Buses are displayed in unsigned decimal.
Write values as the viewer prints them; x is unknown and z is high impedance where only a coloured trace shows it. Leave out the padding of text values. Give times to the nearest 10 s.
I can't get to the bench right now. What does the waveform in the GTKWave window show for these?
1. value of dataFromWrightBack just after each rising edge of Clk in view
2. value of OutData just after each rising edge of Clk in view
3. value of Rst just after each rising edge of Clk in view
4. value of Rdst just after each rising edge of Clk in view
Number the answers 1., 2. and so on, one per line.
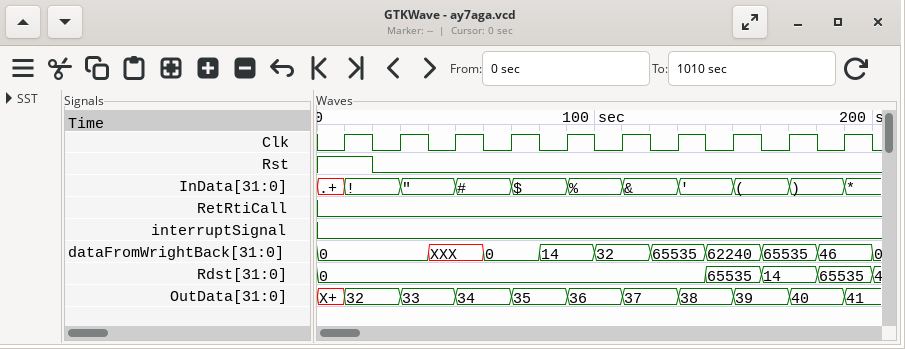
1. 0, 0, XXX, 0, 14, 32, 65535, 62240, 65535, 46
2. 32, 33, 34, 35, 36, 37, 38, 39, 40, 41
3. 1 0 0 0 0 0 0 0 0 0
4. 0, 0, 0, 0, 0, 0, 0, 65535, 14, 65535
